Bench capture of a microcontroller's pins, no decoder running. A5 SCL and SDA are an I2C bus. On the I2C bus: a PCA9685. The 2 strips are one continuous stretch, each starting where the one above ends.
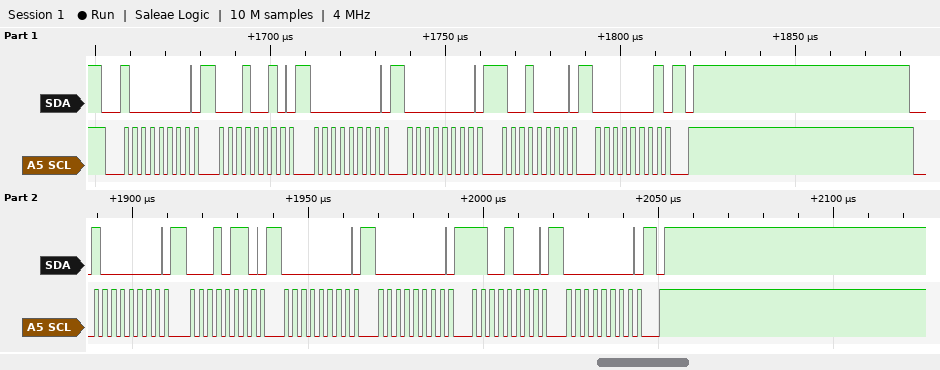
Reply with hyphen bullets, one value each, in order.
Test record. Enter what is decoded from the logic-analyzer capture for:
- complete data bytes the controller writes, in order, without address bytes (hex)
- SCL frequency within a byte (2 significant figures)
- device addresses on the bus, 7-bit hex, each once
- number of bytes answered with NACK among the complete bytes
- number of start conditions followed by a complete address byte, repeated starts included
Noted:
- 12 00 00 90 01 16 00 00 C8 00
- 400 kHz
- 0x40
- 0
- 2
